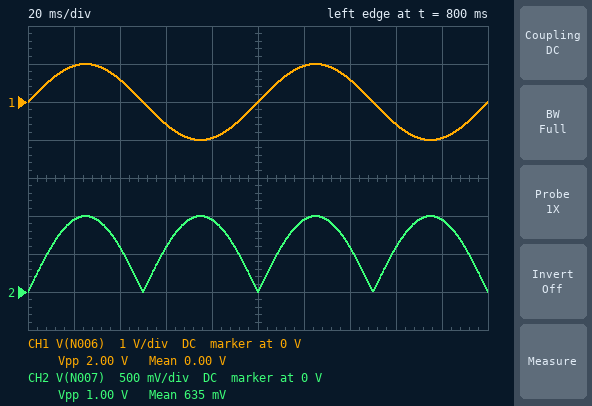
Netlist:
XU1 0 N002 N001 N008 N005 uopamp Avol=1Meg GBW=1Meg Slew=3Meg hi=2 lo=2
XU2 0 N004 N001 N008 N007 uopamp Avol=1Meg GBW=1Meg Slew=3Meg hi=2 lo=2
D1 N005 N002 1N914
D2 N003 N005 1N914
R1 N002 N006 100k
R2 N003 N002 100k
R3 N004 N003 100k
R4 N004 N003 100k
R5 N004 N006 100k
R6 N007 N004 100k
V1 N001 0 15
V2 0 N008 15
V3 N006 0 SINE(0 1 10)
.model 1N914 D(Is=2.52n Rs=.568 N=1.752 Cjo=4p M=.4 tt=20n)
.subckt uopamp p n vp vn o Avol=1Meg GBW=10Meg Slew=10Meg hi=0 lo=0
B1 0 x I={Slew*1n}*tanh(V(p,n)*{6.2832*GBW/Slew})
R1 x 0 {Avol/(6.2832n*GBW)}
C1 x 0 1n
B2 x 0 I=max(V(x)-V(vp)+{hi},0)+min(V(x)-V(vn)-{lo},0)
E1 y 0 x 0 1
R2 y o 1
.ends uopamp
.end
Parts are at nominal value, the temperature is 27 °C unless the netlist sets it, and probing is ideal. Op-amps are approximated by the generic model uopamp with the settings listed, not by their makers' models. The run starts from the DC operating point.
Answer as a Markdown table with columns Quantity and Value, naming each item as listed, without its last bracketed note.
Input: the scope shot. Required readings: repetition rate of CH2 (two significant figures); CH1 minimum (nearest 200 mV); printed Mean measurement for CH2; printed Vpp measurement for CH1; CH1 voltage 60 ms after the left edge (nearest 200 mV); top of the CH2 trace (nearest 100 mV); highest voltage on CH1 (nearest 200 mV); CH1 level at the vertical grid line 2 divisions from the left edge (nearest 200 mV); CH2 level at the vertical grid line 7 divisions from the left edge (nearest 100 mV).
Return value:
| Quantity | Value |
|---|---|
| repetition rate of CH2 | 20 Hz |
| CH1 minimum | -1.0 V |
| printed Mean measurement for CH2 | 635 mV |
| printed Vpp measurement for CH1 | 2.00 V |
| CH1 voltage 60 ms after the left edge | -600 mV |
| top of the CH2 trace | 1.0 V |
| highest voltage on CH1 | 1.0 V |
| CH1 level at the vertical grid line 2 divisions from the left edge | 600 mV |
| CH2 level at the vertical grid line 7 divisions from the left edge | 600 mV |
